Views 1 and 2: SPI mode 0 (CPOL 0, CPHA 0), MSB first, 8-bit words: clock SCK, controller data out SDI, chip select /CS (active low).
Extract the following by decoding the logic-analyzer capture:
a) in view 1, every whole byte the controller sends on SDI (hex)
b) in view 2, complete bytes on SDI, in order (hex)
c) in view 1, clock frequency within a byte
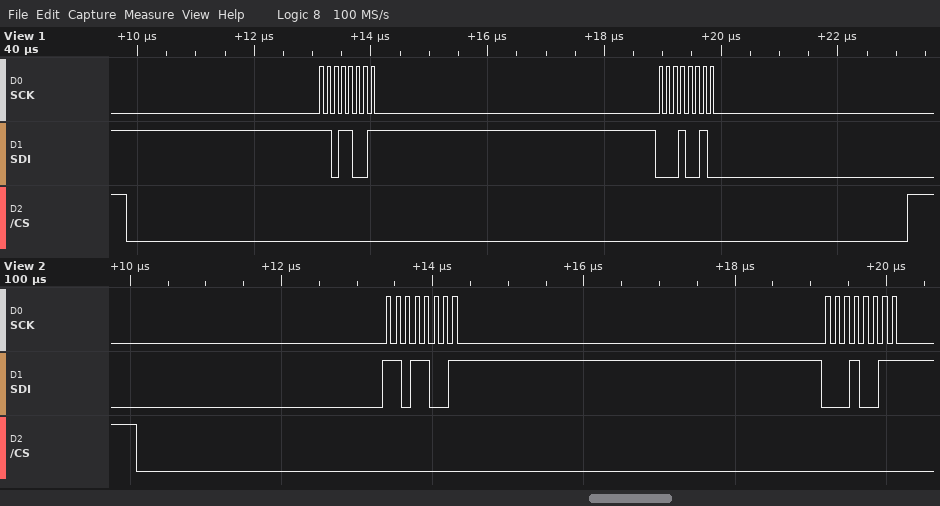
D9 12
D9 13
8 MHz
